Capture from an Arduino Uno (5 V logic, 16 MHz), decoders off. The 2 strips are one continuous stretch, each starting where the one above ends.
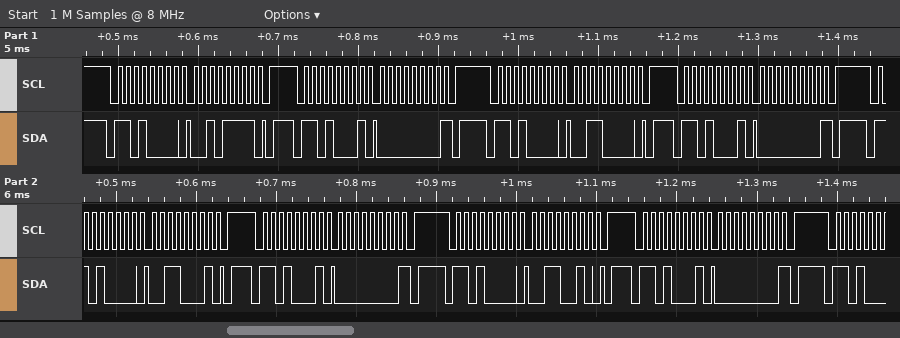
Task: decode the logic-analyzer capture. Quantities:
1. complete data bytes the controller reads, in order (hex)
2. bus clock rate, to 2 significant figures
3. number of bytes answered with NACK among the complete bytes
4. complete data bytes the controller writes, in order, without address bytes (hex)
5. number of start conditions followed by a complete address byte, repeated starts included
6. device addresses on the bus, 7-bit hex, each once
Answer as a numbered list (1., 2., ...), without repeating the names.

1. 00 00 00 00
2. 100 kHz
3. 4
4. 2F 30 31 32
5. 8
6. 0x68
